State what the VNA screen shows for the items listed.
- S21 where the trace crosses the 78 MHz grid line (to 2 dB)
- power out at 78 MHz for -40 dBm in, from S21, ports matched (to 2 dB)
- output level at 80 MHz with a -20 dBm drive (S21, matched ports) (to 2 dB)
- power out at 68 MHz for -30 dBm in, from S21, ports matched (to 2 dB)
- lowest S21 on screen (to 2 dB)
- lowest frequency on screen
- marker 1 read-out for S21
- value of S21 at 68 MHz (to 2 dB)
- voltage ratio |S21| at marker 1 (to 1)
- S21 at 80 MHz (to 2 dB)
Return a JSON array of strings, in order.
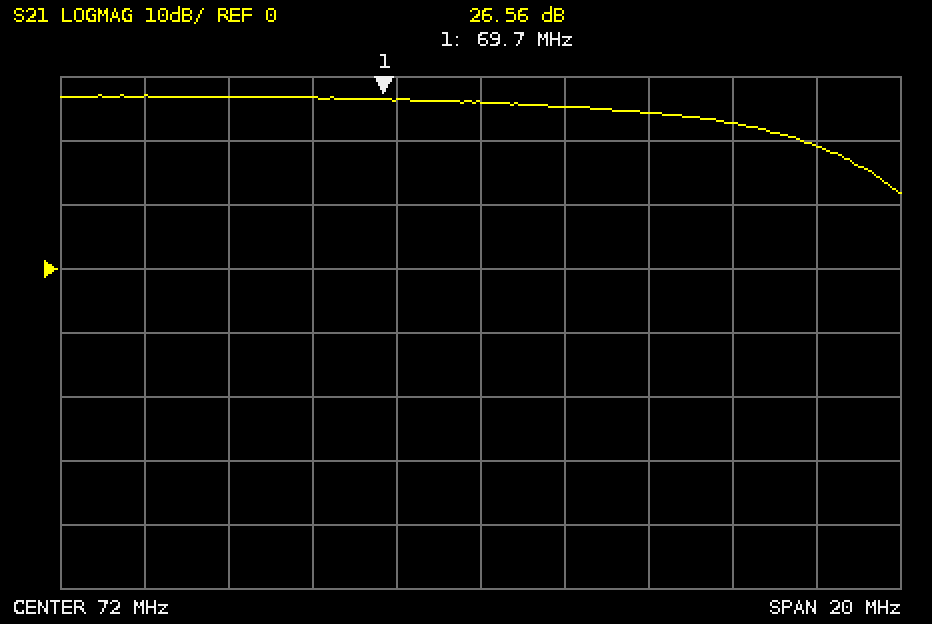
["22 dB", "-18 dBm", "0 dBm", "-4 dBm", "12 dB", "62 MHz", "26.56 dB", "26 dB", "21", "20 dB"]
